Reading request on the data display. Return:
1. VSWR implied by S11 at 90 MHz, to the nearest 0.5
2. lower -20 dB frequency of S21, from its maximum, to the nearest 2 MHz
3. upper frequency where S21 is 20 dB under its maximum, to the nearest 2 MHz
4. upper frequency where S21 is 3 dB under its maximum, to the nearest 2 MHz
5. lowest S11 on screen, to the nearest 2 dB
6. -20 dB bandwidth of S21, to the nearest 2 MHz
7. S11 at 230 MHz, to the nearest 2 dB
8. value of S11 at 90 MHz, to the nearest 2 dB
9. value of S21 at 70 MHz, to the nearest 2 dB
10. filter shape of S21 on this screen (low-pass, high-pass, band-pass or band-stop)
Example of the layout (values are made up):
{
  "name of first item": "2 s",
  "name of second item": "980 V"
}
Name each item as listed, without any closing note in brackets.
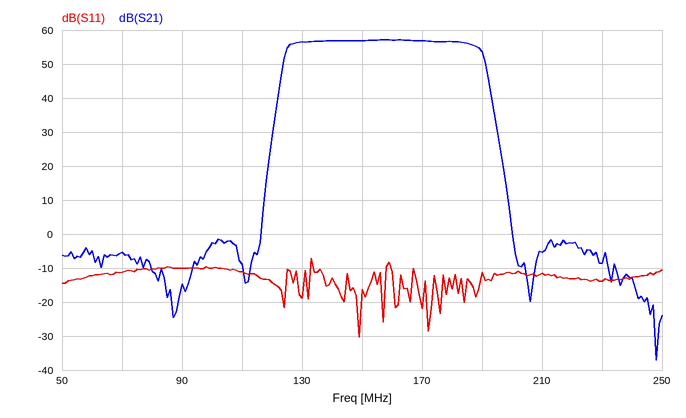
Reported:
{
  "VSWR implied by S11 at 90 MHz, to the nearest 0.5": "2.0",
  "lower -20 dB frequency of S21, from its maximum, to the nearest 2 MHz": "122 MHz",
  "upper frequency where S21 is 20 dB under its maximum, to the nearest 2 MHz": "194 MHz",
  "upper frequency where S21 is 3 dB under its maximum, to the nearest 2 MHz": "190 MHz",
  "lowest S11 on screen, to the nearest 2 dB": "-30 dB",
  "-20 dB bandwidth of S21, to the nearest 2 MHz": "72 MHz",
  "S11 at 230 MHz, to the nearest 2 dB": "-14 dB",
  "value of S11 at 90 MHz, to the nearest 2 dB": "-10 dB",
  "value of S21 at 70 MHz, to the nearest 2 dB": "-6 dB",
  "filter shape of S21 on this screen": "band-pass"
}
